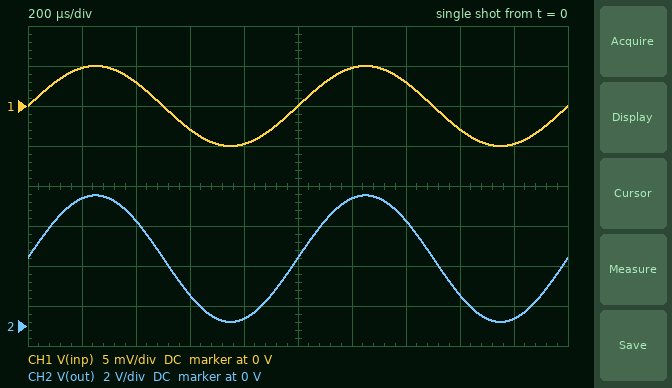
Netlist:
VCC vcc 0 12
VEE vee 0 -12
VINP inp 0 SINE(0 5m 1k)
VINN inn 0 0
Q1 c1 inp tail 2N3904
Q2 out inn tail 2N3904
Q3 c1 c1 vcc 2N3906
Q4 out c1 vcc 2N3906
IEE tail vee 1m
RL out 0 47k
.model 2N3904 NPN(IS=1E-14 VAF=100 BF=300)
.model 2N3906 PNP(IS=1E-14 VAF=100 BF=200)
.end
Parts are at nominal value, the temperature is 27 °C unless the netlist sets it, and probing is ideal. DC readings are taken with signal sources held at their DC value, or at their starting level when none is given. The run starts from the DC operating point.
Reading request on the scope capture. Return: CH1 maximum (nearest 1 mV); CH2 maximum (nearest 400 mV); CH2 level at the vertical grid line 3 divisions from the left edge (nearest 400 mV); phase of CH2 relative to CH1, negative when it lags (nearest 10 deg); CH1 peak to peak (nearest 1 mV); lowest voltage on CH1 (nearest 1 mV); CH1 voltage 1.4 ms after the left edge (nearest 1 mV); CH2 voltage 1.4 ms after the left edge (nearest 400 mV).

5 mV
6.4 V
1.6 V
0 deg
10 mV
-5 mV
3 mV
5.2 V
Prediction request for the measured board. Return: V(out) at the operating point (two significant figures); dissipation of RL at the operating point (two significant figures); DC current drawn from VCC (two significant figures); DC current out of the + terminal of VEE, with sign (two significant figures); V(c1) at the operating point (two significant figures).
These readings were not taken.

3.4 V
250 µW
1.1 mA
-1.0 mA
11 V
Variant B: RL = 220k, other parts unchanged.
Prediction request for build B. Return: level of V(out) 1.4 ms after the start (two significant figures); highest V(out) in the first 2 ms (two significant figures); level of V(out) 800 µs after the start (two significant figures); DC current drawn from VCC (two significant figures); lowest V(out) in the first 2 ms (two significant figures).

11 V
12 V
780 mV
1.0 mA
440 mV
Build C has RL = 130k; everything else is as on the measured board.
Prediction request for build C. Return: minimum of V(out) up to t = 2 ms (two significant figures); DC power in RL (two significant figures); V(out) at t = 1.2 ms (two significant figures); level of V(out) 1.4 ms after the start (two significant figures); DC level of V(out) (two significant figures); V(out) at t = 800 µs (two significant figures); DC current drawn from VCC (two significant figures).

360 mV
280 µW
11 V
9.3 V
6.0 V
640 mV
1.0 mA
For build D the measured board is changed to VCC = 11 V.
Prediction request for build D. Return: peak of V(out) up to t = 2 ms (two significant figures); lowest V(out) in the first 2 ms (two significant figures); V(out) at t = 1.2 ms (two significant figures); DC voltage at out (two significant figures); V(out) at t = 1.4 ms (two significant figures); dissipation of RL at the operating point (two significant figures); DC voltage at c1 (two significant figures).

6.2 V
-100 mV
6.1 V
3.1 V
4.9 V
200 µW
10 V
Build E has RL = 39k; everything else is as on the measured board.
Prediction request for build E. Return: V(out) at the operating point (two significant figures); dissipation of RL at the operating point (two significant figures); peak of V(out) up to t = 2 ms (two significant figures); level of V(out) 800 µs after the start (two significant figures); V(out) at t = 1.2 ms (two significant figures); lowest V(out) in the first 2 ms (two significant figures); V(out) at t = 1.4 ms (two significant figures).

3.0 V
230 µW
5.7 V
320 mV
5.6 V
180 mV
4.6 V
